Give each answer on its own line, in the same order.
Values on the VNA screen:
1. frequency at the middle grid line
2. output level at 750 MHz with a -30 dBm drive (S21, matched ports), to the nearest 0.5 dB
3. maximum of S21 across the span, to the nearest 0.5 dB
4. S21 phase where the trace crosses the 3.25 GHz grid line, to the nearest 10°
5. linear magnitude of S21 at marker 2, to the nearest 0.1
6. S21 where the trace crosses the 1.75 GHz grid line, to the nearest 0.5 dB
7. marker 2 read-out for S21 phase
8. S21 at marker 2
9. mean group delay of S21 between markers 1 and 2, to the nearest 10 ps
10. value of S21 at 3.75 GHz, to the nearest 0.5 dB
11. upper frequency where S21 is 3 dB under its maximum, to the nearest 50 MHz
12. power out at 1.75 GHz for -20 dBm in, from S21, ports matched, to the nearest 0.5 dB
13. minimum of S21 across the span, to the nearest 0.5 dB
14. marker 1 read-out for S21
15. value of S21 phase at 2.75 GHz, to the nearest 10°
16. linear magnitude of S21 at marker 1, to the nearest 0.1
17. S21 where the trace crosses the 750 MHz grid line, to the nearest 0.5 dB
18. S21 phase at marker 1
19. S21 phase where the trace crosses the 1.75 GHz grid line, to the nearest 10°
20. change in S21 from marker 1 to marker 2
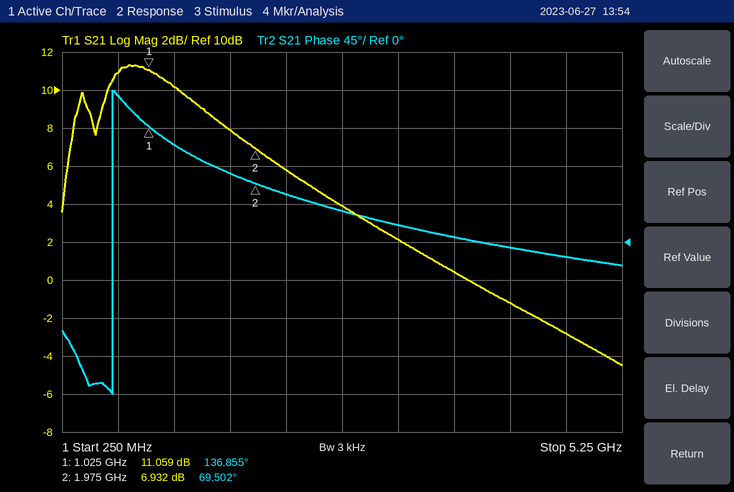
2.75 GHz
-19.0 dBm
11.5 dB
20°
2.2
8.0 dB
69.502°
6.932 dB
200 ps
0.5 dB
1.65 GHz
-12.0 dBm
-4.5 dB
11.059 dB
40°
3.6
11.0 dB
136.855°
80°
-4.127 dB
